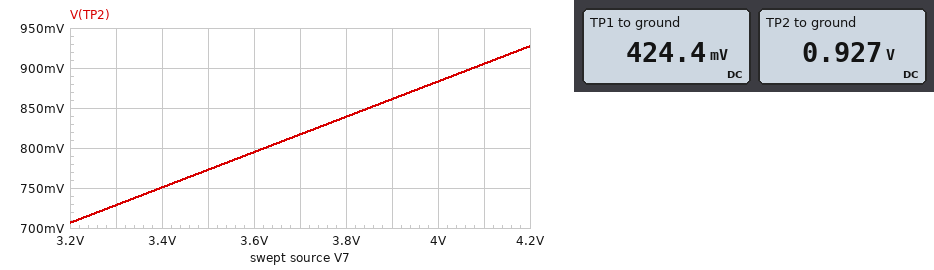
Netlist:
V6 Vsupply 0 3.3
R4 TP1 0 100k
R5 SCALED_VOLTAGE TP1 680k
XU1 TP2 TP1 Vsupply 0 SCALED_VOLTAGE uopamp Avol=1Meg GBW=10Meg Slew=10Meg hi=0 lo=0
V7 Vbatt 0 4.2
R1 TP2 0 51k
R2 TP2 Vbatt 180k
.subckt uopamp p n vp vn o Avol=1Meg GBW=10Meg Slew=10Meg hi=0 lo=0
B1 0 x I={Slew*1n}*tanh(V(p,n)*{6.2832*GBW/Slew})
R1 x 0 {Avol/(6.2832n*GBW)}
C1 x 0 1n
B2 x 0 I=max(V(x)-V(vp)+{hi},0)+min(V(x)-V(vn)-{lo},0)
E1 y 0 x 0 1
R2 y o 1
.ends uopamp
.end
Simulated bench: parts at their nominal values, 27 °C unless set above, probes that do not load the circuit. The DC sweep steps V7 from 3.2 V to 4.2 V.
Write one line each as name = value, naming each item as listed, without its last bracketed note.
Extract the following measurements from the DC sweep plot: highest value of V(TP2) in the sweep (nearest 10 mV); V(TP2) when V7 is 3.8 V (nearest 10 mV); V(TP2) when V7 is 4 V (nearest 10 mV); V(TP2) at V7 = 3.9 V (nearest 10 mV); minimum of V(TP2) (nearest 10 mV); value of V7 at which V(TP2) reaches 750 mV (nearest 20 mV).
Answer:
highest value of V(TP2) in the sweep = 930 mV
V(TP2) when V7 is 3.8 V = 840 mV
V(TP2) when V7 is 4 V = 880 mV
V(TP2) at V7 = 3.9 V = 860 mV
minimum of V(TP2) = 710 mV
value of V7 at which V(TP2) reaches 750 mV = 3.40 V
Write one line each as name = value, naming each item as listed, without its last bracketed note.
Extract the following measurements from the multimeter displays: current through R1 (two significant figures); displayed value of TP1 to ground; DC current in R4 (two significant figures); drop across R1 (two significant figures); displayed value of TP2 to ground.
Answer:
current through R1 = 18 µA
displayed value of TP1 to ground = 424.4 mV
DC current in R4 = 4.2 µA
drop across R1 = 930 mV
displayed value of TP2 to ground = 0.927 V
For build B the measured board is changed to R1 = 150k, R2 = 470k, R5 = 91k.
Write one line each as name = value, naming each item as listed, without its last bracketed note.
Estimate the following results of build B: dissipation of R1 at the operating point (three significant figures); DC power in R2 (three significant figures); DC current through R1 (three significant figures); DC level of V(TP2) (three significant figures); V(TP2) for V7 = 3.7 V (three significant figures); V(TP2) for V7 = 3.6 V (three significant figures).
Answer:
dissipation of R1 at the operating point = 6.88 µW
DC power in R2 = 21.6 µW
DC current through R1 = 6.77 µA
DC level of V(TP2) = 1.02 V
V(TP2) for V7 = 3.7 V = 895 mV
V(TP2) for V7 = 3.6 V = 871 mV
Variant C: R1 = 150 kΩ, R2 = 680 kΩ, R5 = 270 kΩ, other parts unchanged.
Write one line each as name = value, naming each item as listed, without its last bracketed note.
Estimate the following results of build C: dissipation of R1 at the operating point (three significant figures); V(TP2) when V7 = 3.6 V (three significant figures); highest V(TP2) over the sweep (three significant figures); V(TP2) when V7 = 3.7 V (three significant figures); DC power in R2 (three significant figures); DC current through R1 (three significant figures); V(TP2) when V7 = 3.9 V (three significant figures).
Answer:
dissipation of R1 at the operating point = 3.84 µW
V(TP2) when V7 = 3.6 V = 651 mV
highest V(TP2) over the sweep = 759 mV
V(TP2) when V7 = 3.7 V = 669 mV
DC power in R2 = 17.4 µW
DC current through R1 = 5.06 µA
V(TP2) when V7 = 3.9 V = 705 mV
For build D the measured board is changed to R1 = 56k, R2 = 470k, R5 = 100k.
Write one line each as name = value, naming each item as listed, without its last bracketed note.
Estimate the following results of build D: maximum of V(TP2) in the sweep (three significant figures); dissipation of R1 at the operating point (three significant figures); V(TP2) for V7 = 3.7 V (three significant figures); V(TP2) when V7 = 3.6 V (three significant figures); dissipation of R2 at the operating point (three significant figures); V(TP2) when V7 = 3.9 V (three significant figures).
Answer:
maximum of V(TP2) in the sweep = 447 mV
dissipation of R1 at the operating point = 3.57 µW
V(TP2) for V7 = 3.7 V = 394 mV
V(TP2) when V7 = 3.6 V = 383 mV
dissipation of R2 at the operating point = 30.0 µW
V(TP2) when V7 = 3.9 V = 415 mV
